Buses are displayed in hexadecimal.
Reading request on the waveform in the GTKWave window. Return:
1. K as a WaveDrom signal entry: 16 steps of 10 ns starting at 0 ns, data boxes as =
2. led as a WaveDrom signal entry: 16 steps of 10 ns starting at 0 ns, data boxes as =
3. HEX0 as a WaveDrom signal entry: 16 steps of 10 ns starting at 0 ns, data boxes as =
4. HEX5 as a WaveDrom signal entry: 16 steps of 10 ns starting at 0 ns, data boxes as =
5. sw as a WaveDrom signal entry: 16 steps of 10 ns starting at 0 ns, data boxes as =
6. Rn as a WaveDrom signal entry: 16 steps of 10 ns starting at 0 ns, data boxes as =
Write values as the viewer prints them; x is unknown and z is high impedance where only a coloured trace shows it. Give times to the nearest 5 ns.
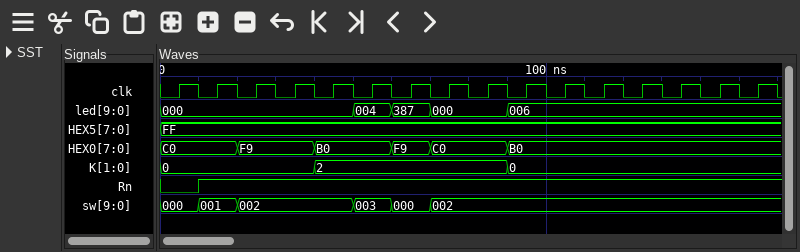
{name: 'K', wave: '=...=....=......', data: '0 2 0'}
{name: 'led', wave: '=....===.=......', data: '000 004 387 000 006'}
{name: 'HEX0', wave: '=.=.=.==.=......', data: 'C0 F9 B0 F9 C0 B0'}
{name: 'HEX5', wave: '=...............', data: 'FF'}
{name: 'sw', wave: '===..===........', data: '000 001 002 003 000 002'}
{name: 'Rn', wave: '01..............'}
